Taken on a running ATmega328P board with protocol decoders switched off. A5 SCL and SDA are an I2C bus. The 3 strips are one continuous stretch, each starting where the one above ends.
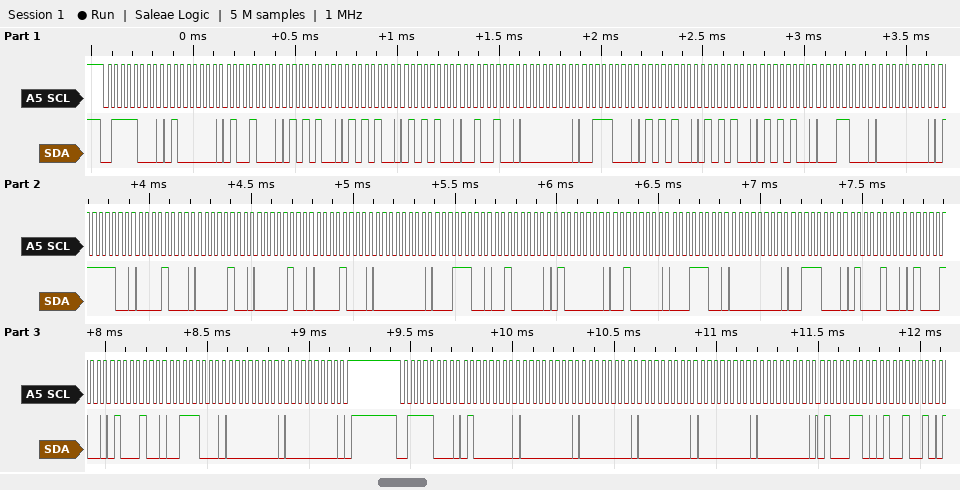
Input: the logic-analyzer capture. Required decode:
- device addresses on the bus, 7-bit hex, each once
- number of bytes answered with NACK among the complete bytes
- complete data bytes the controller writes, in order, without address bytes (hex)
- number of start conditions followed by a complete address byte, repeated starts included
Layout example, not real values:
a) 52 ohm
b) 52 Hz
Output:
a) 0x3C
b) 0
c) 40 48 54 54 54 24 00 38 54 54 54 18 00 7C 08 04 04 08 00 1C 20 40 20 1C 00 38 44 44 44 38 00 00 40 00 00 00 00 00 46 49
d) 2
